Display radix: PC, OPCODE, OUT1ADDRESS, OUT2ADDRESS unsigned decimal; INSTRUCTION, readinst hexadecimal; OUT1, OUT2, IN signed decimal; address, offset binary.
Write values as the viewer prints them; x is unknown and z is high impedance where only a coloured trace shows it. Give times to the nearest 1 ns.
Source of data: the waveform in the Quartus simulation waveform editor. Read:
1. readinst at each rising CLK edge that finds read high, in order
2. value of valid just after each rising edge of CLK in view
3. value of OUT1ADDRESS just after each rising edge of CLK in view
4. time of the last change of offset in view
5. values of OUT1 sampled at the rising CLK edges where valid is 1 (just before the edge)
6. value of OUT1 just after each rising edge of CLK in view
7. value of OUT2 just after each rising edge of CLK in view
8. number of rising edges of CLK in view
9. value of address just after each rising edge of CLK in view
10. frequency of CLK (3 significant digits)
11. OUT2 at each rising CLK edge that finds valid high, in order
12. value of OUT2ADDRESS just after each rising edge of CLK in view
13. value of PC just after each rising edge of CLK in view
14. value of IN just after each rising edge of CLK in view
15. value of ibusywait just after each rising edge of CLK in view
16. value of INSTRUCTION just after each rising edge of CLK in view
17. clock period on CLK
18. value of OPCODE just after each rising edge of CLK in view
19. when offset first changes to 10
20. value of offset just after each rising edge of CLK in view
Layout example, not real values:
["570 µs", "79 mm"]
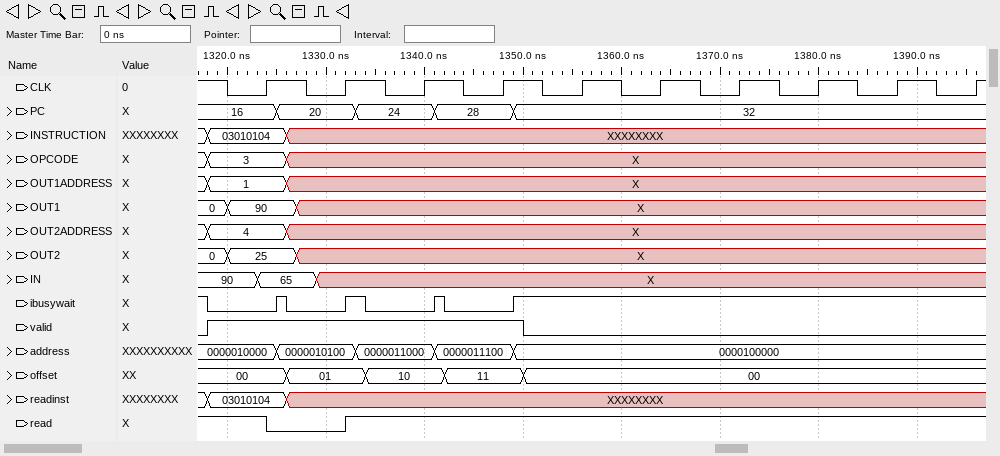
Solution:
["03010104, XXXXXXXX, XXXXXXXX, XXXXXXXX, XXXXXXXX, XXXXXXXX, XXXXXXXX, XXXXXXXX, XXXXXXXX", "1 1 1 1 0 0 0 0 0 0", "1, X, X, X, X, X, X, X, X, X", "1350 ns", "90, X, X, X", "90, X, X, X, X, X, X, X, X, X", "25, X, X, X, X, X, X, X, X, X", "10", "0000010000, 0000010100, 0000011000, 0000011100, 0000100000, 0000100000, 0000100000, 0000100000, 0000100000, 0000100000", "125 MHz", "25, X, X, X", "4, X, X, X, X, X, X, X, X, X", "16, 20, 24, 28, 32, 32, 32, 32, 32, 32", "65, X, X, X, X, X, X, X, X, X", "0 1 0 0 1 1 1 1 1 1", "03010104, XXXXXXXX, XXXXXXXX, XXXXXXXX, XXXXXXXX, XXXXXXXX, XXXXXXXX, XXXXXXXX, XXXXXXXX, XXXXXXXX", "8 ns", "3, X, X, X, X, X, X, X, X, X", "1334 ns", "00, 01, 10, 11, 00, 00, 00, 00, 00, 00"]
